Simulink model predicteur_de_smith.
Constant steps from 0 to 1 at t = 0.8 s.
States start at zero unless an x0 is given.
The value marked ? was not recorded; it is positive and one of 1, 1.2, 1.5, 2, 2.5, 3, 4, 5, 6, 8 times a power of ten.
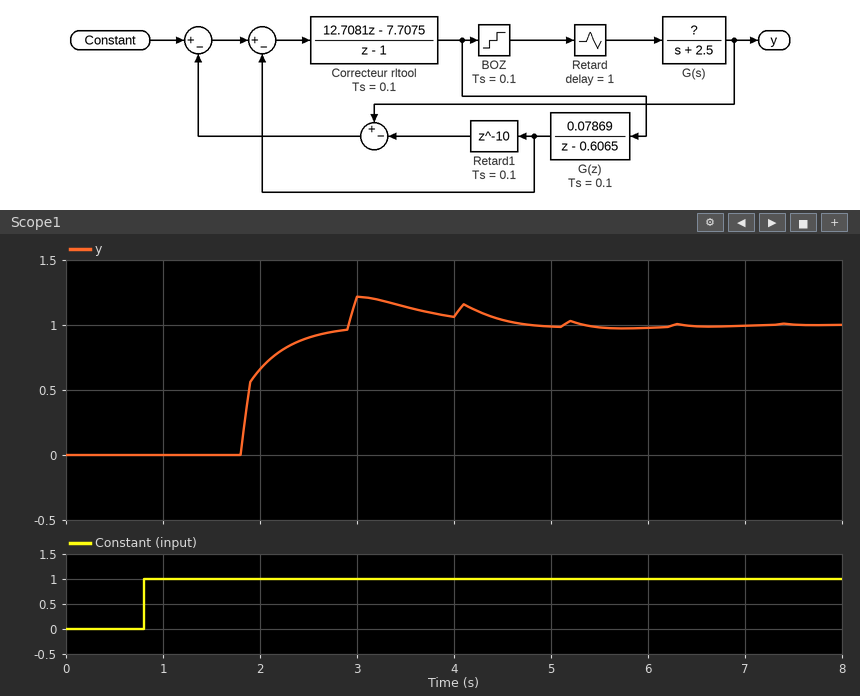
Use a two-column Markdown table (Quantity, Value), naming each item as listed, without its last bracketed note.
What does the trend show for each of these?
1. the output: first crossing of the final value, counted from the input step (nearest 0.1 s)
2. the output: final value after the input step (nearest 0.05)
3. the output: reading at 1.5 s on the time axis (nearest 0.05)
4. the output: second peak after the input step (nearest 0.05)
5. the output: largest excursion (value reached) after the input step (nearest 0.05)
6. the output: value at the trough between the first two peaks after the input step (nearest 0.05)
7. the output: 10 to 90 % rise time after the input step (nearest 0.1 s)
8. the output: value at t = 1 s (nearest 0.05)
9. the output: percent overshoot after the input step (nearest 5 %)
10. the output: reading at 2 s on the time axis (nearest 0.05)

| Quantity | Value |
|---|---|
| the output: first crossing of the final value, counted from the input step | 2.1 s |
| the output: final value after the input step | 1.00 |
| the output: reading at 1.5 s on the time axis | 0.00 |
| the output: second peak after the input step | 1.15 |
| the output: largest excursion (value reached) after the input step | 1.20 |
| the output: value at the trough between the first two peaks after the input step | 1.05 |
| the output: 10 to 90 % rise time after the input step | 0.7 s |
| the output: value at t = 1 s | 0.00 |
| the output: percent overshoot after the input step | 20 % |
| the output: reading at 2 s on the time axis | 0.65 |
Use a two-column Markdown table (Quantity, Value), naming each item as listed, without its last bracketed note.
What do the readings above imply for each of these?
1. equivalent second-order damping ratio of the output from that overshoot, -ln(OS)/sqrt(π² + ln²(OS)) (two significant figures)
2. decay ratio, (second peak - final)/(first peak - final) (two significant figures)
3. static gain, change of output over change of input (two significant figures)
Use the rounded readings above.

| Quantity | Value |
|---|---|
| equivalent second-order damping ratio of the output from that overshoot, -ln(OS)/sqrt(π² + ln²(OS)) | 0.46 |
| decay ratio, (second peak - final)/(first peak - final) | 0.75 |
| static gain, change of output over change of input | 1.0 |
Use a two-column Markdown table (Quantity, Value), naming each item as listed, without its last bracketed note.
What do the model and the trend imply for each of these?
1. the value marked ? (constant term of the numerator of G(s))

| Quantity | Value |
|---|---|
| the value marked ? (constant term of the numerator of G(s)) | 0.5 |
